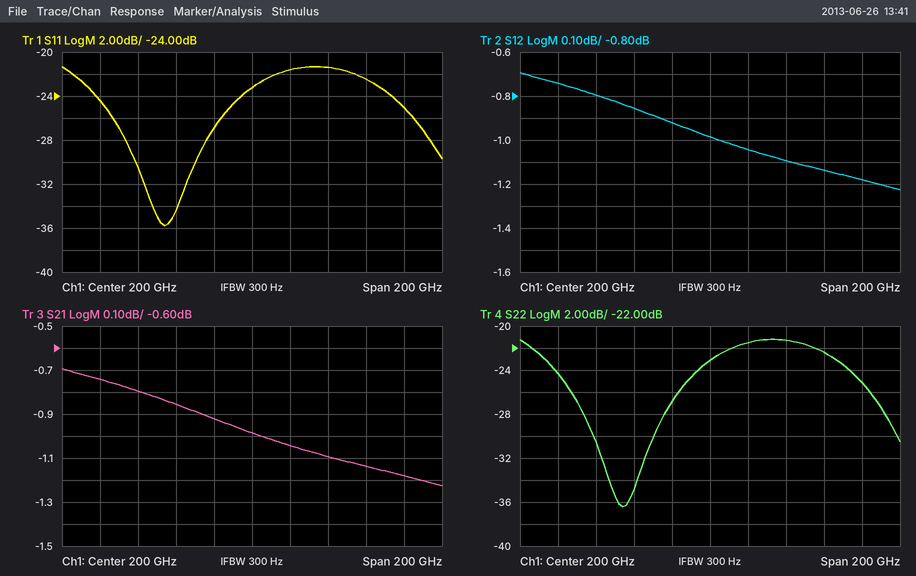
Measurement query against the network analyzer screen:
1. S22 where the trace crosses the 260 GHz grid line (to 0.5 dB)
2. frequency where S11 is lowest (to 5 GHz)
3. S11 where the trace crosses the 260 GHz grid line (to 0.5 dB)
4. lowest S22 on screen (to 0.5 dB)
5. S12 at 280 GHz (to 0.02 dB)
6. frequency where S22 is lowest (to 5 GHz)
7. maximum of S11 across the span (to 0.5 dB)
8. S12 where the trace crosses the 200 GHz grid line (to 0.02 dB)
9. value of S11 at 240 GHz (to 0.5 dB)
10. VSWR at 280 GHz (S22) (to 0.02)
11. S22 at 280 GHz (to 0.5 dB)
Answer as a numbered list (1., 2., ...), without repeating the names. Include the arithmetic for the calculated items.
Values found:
1. -22.5 dB
2. 155 GHz
3. -22.5 dB
4. -36.5 dB
5. -1.18 dB
6. 155 GHz
7. -21.5 dB
8. -0.98 dB
9. -21.5 dB
10. |Γ| = 10^(-25/20) = 0.0562; VSWR = (1 + 0.0562)/(1 − 0.0562) ≈ 1.12
11. -25.0 dB
